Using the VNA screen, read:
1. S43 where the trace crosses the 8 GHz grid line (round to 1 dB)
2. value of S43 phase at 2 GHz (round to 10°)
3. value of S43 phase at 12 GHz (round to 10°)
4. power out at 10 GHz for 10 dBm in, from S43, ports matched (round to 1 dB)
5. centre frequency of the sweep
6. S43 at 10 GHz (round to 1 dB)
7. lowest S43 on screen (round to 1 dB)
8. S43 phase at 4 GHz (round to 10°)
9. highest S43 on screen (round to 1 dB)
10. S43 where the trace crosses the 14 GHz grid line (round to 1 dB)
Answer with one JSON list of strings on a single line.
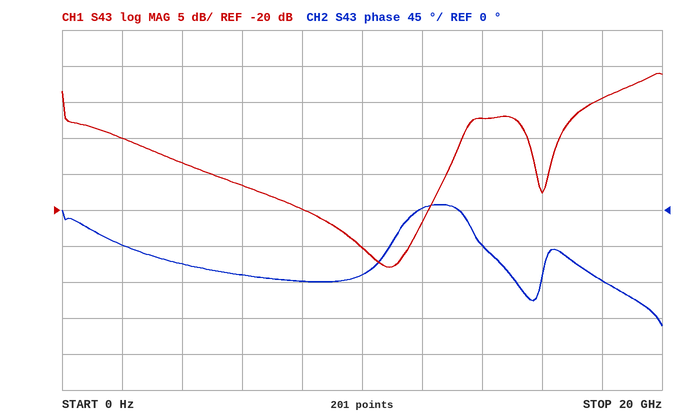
["-20 dB", "-40°", "0°", "-15 dBm", "10 GHz", "-25 dB", "-28 dB", "-70°", "-1 dB", "-7 dB"]
